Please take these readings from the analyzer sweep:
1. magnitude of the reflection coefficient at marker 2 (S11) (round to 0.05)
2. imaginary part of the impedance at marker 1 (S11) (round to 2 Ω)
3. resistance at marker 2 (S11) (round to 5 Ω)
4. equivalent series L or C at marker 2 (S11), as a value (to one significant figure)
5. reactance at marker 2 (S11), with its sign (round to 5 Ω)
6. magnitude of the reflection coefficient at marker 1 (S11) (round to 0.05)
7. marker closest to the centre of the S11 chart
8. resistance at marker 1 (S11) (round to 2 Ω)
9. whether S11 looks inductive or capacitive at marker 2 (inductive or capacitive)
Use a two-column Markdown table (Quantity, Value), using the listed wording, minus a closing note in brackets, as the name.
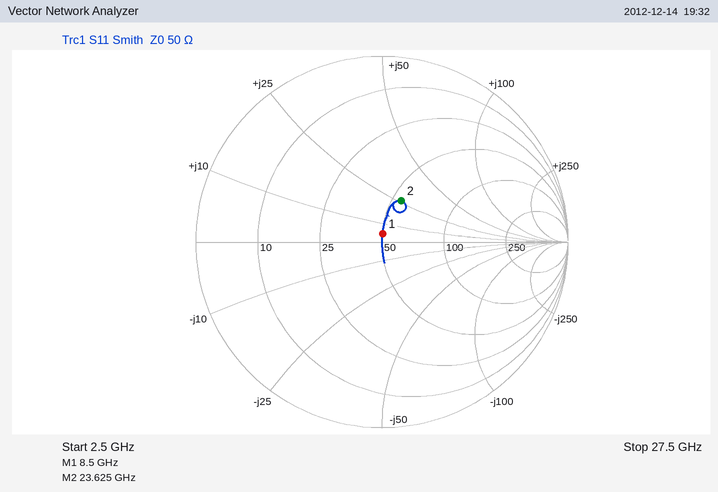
| Quantity | Value |
|---|---|
| magnitude of the reflection coefficient at marker 2 (S11) | 0.25 |
| imaginary part of the impedance at marker 1 (S11) | +4 Ω |
| resistance at marker 2 (S11) | 55 Ω |
| equivalent series L or C at marker 2 (S11), as a value | 200 pH |
| reactance at marker 2 (S11), with its sign | +25 Ω |
| magnitude of the reflection coefficient at marker 1 (S11) | 0.05 |
| marker closest to the centre of the S11 chart | marker 1 |
| resistance at marker 1 (S11) | 50 Ω |
| whether S11 looks inductive or capacitive at marker 2 | inductive |
